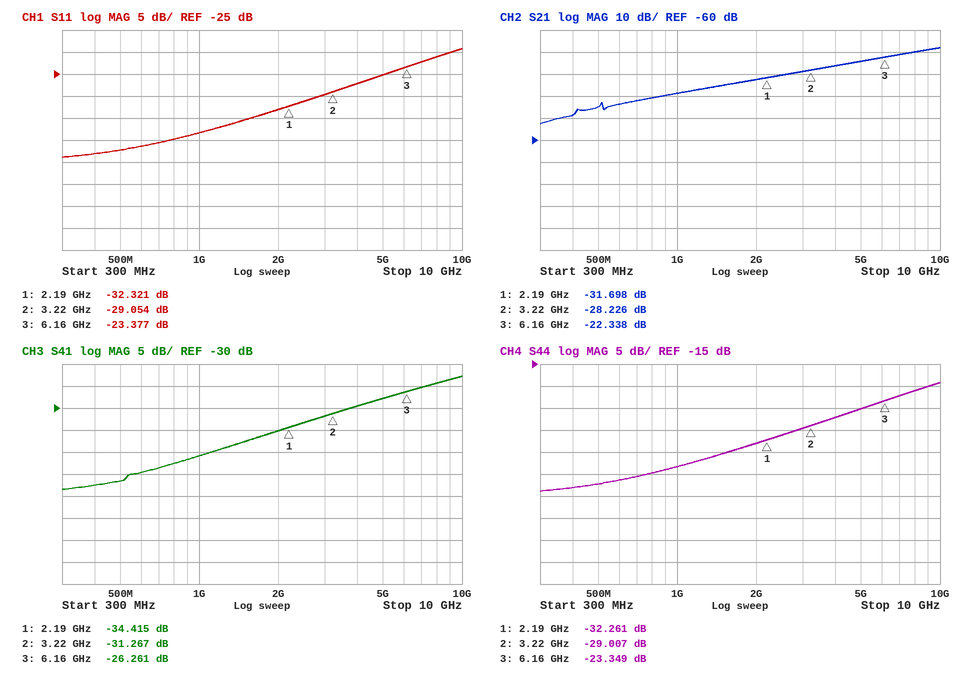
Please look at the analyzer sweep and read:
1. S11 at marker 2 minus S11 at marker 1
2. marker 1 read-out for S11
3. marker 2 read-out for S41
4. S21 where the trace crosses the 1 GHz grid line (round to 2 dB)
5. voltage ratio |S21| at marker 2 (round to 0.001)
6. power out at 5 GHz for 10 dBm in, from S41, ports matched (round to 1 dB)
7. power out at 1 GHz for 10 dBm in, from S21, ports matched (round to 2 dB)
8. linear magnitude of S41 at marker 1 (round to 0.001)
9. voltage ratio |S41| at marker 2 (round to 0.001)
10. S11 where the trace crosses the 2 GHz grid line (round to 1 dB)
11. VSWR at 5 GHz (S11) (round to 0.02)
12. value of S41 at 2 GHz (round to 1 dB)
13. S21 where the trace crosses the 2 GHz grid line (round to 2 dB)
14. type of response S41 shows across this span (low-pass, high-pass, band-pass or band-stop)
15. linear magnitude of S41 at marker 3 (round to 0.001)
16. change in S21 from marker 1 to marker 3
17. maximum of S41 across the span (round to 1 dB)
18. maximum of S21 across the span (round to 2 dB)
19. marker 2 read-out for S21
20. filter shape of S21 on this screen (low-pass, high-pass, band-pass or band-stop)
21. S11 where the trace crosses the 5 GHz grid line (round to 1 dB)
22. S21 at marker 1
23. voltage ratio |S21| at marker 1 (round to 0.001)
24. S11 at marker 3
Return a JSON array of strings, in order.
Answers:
["3.267 dB", "-32.321 dB", "-31.267 dB", "-38 dB", "0.039", "-18 dBm", "-28 dBm", "0.019", "0.027", "-33 dB", "1.12", "-35 dB", "-32 dB", "high-pass", "0.049", "9.360 dB", "-23 dB", "-18 dB", "-28.226 dB", "high-pass", "-25 dB", "-31.698 dB", "0.026", "-23.377 dB"]
